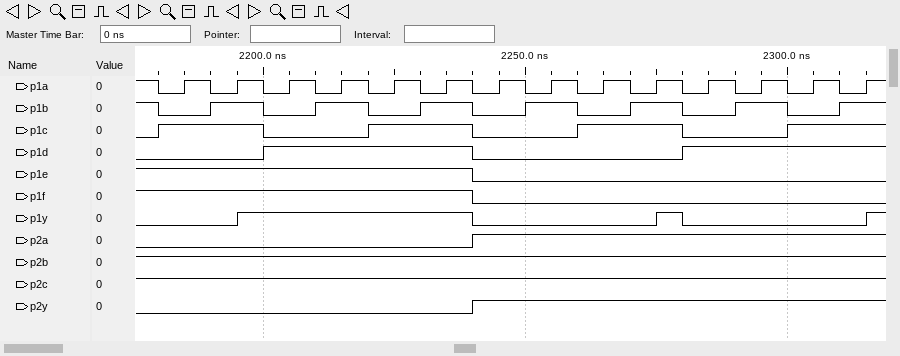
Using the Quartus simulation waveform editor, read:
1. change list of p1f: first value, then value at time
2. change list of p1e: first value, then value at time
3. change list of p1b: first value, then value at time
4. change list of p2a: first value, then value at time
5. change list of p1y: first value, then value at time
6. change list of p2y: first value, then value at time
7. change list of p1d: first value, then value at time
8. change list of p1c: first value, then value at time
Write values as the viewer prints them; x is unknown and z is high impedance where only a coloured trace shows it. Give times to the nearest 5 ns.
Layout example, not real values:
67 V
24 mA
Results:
1, 0 at 2240 ns
1, 0 at 2240 ns
1, 0 at 2180 ns, 1 at 2190 ns, 0 at 2200 ns, 1 at 2210 ns, 0 at 2220 ns, 1 at 2230 ns, 0 at 2240 ns, 1 at 2250 ns, 0 at 2260 ns, 1 at 2270 ns, 0 at 2280 ns, 1 at 2290 ns, 0 at 2300 ns, 1 at 2310 ns
0, 1 at 2240 ns
0, 1 at 2195 ns, 0 at 2240 ns, 1 at 2275 ns, 0 at 2280 ns, 1 at 2315 ns
0, 1 at 2240 ns
0, 1 at 2200 ns, 0 at 2240 ns, 1 at 2280 ns
0, 1 at 2180 ns, 0 at 2200 ns, 1 at 2220 ns, 0 at 2240 ns, 1 at 2260 ns, 0 at 2280 ns, 1 at 2300 ns
